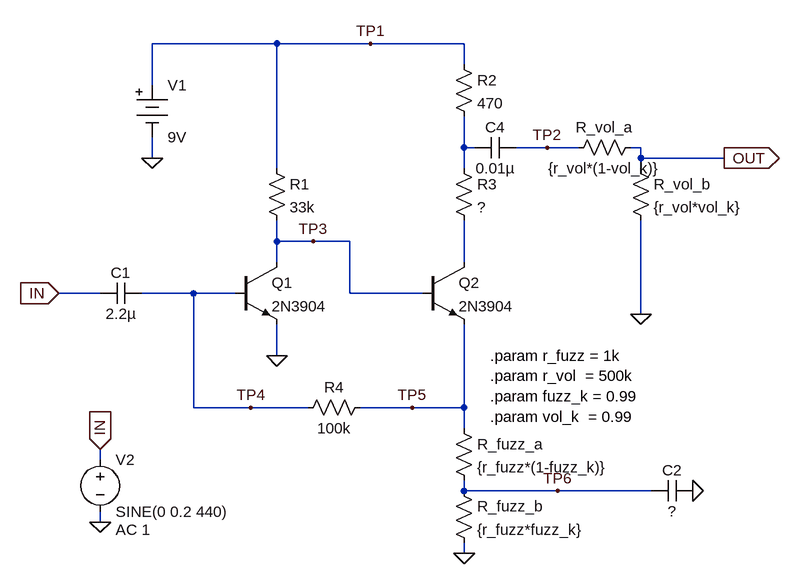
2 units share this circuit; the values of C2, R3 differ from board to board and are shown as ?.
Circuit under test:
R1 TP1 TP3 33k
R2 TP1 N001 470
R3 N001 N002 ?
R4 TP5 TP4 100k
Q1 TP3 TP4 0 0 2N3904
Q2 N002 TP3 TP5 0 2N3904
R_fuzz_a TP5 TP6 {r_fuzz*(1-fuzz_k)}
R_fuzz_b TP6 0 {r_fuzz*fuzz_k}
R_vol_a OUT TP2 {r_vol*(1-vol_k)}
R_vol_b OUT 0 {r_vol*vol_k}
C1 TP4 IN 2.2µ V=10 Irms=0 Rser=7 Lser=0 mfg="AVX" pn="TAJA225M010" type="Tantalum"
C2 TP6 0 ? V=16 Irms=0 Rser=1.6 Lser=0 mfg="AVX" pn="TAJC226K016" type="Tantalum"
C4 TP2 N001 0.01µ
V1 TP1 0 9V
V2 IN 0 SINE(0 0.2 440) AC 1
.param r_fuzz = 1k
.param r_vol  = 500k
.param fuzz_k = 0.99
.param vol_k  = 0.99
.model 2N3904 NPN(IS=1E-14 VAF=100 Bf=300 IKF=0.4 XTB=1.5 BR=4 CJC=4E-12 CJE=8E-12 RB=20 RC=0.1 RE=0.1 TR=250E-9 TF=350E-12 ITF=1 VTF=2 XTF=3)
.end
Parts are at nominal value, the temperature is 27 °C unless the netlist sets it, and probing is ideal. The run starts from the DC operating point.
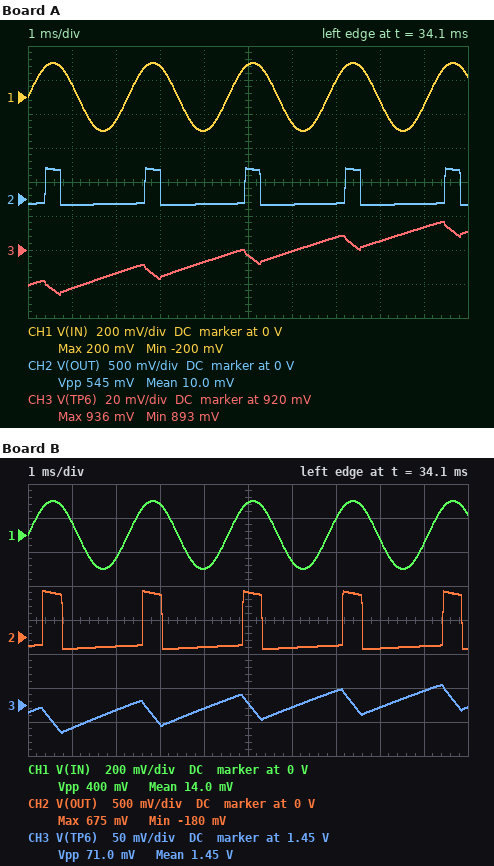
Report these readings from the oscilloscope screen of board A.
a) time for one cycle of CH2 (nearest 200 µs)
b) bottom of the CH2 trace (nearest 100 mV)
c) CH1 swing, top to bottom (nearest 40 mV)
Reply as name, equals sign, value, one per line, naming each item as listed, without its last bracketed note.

time for one cycle of CH2 = 2.2 ms
bottom of the CH2 trace = -100 mV
CH1 swing, top to bottom = 400 mV
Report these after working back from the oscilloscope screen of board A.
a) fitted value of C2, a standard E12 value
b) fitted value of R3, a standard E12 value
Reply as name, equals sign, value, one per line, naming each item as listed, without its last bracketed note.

fitted value of C2, a standard E12 value = 47 µF
fitted value of R3, a standard E12 value = 6.8 kΩ
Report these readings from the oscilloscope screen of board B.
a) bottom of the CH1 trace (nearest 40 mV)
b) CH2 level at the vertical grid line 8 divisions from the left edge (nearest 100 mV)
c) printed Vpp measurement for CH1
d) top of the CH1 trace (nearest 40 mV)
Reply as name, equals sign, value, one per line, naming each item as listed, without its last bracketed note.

bottom of the CH1 trace = -200 mV
CH2 level at the vertical grid line 8 divisions from the left edge = -200 mV
printed Vpp measurement for CH1 = 400 mV
top of the CH1 trace = 200 mV
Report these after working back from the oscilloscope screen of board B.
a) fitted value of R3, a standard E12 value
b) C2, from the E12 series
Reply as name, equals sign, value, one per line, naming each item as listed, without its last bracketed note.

fitted value of R3, a standard E12 value = 3.9 kΩ
C2, from the E12 series = 18 µF
